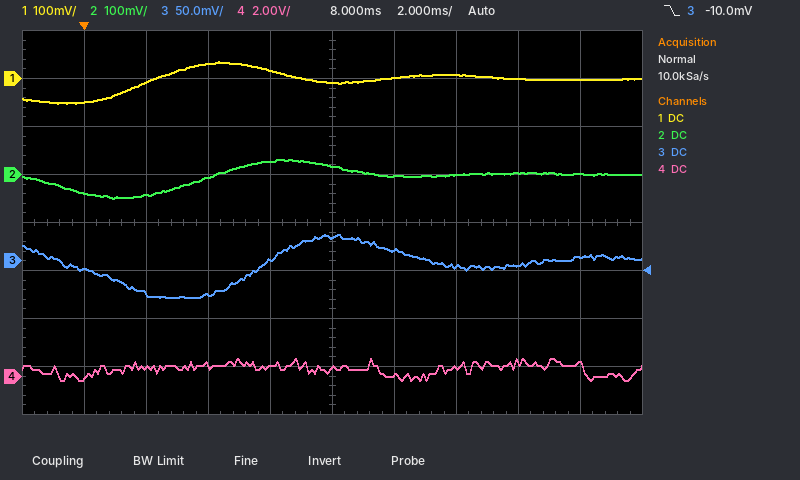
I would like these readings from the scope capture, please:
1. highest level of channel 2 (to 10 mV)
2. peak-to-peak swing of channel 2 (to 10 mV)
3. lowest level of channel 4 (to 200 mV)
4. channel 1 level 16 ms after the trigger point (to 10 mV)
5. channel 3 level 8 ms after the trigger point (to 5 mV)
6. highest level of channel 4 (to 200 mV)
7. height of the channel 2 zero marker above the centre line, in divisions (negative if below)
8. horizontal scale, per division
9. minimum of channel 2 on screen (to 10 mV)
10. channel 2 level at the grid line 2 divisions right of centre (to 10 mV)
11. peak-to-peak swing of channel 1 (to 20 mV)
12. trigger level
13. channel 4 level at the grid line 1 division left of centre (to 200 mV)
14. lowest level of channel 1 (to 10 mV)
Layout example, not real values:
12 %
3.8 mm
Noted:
30 mV
80 mV
-200 mV
0 mV
25 mV
800 mV
+1.0 div
2 ms
-50 mV
0 mV
80 mV
-10.0 mV
400 mV
-50 mV
